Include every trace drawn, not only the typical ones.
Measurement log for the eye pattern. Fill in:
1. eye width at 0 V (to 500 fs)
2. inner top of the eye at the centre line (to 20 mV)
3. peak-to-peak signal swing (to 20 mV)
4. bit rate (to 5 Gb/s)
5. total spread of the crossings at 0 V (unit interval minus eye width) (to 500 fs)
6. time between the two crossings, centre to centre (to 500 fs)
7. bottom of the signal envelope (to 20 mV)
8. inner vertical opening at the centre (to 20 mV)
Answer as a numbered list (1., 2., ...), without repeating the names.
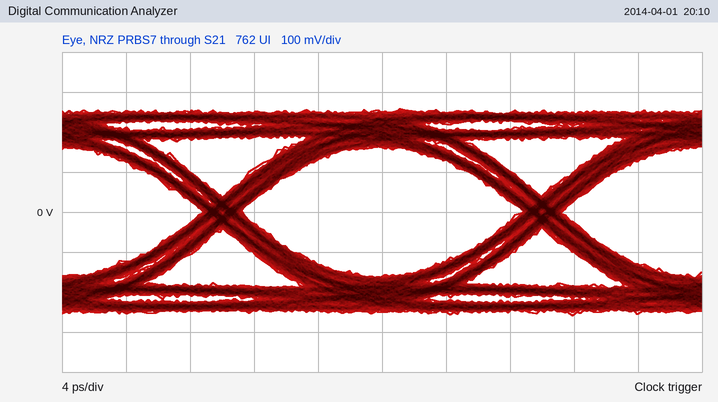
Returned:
1. 17.5 ps
2. 160 mV
3. 520 mV
4. 50 Gb/s
5. 2.5 ps
6. 20.0 ps
7. -260 mV
8. 320 mV
